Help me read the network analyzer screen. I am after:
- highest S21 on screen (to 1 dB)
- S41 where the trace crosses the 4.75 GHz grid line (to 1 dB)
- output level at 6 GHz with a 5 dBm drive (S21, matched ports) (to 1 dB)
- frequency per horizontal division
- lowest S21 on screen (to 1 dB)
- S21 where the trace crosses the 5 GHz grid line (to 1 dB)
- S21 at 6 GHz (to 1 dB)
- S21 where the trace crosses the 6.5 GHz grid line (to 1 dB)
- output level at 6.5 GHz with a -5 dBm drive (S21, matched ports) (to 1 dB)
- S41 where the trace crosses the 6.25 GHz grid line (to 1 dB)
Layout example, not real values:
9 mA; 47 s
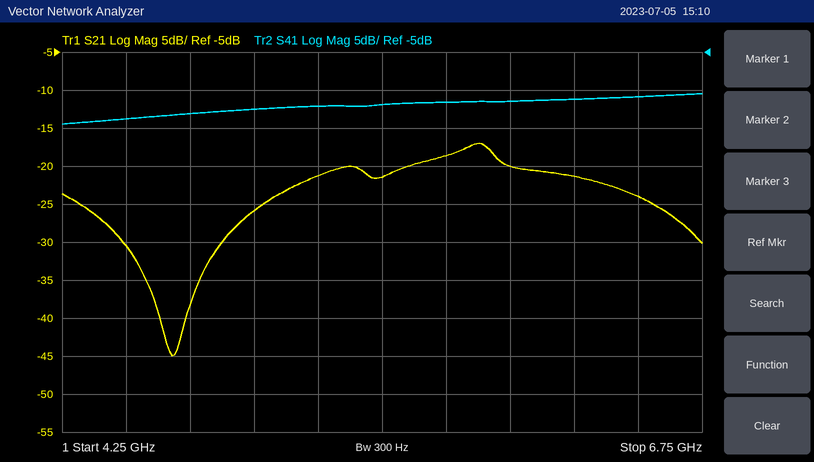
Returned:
-17 dB; -13 dB; -15 dBm; 250 MHz; -45 dB; -26 dB; -20 dB; -24 dB; -29 dBm; -11 dB
